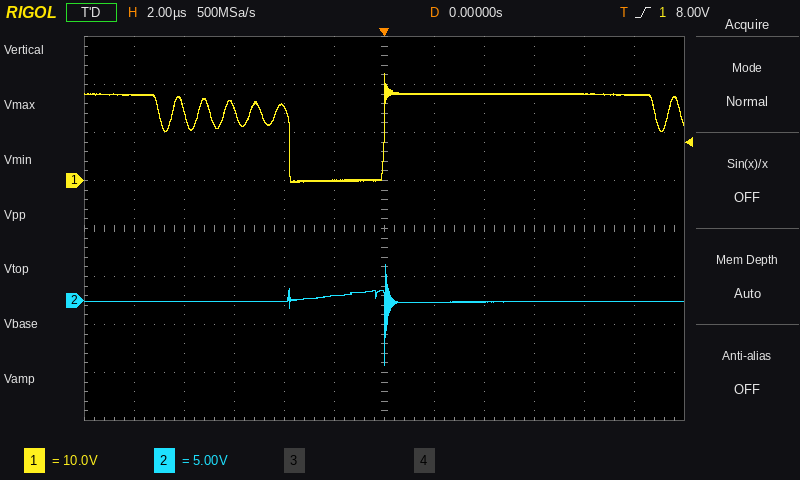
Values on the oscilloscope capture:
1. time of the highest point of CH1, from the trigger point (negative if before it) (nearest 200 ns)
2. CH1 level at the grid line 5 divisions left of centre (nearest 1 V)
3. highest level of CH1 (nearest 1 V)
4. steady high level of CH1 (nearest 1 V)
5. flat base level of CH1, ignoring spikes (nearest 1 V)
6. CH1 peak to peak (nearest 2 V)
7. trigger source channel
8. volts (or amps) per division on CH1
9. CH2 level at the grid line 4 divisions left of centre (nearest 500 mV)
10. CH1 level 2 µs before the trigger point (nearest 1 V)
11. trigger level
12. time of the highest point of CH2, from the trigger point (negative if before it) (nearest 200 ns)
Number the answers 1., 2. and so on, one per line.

1. 0.0 µs
2. 18 V
3. 22 V
4. 18 V
5. 0 V
6. 22 V
7. CH1
8. 10 V
9. 0.0 V
10. 0 V
11. 8.00 V
12. 0.0 µs
